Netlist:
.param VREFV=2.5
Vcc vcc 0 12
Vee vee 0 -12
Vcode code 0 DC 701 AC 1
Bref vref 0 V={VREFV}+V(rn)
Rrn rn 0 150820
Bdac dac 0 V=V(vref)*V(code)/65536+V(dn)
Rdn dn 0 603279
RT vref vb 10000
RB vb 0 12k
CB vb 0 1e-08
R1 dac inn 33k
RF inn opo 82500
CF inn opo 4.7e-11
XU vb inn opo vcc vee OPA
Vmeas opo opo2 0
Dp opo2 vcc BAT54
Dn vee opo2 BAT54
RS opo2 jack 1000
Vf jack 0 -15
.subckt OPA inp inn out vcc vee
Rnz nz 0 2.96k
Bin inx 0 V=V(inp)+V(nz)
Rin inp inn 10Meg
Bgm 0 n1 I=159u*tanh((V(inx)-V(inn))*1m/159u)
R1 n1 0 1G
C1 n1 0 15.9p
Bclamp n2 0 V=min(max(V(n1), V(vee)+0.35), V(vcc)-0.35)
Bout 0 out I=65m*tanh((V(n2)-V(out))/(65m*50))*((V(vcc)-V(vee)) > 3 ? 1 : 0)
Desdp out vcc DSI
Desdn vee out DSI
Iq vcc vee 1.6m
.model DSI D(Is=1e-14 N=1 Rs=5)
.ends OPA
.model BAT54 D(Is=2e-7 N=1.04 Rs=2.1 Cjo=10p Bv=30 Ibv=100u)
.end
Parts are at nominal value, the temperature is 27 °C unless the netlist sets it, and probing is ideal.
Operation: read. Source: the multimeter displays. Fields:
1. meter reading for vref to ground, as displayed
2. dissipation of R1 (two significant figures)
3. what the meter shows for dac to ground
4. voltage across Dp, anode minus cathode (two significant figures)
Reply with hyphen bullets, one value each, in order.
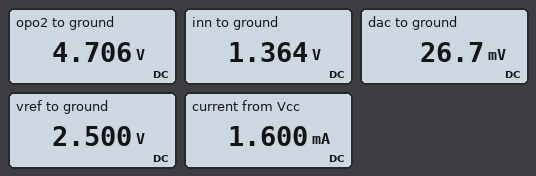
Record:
- 2.500 V
- 54 µW
- 26.7 mV
- -7.3 V
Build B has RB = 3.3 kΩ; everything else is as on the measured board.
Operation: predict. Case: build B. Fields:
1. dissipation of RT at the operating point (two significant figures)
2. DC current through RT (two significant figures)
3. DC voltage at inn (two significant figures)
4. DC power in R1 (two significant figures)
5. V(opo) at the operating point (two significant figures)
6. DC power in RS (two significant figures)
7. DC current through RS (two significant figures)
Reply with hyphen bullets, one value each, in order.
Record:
- 350 µW
- 190 µA
- 620 mV
- 11 µW
- 2.1 V
- 290 mW
- 17 mA
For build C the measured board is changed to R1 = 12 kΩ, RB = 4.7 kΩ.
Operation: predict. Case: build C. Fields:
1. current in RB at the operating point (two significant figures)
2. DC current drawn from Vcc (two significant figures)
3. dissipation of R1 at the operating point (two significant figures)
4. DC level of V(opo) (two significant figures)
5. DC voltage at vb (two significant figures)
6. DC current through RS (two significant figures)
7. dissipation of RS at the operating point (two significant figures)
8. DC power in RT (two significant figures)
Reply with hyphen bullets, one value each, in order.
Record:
- 170 µA
- 1.6 mA
- 50 µW
- 6.1 V
- 800 mV
- 21 mA
- 450 mW
- 290 µW
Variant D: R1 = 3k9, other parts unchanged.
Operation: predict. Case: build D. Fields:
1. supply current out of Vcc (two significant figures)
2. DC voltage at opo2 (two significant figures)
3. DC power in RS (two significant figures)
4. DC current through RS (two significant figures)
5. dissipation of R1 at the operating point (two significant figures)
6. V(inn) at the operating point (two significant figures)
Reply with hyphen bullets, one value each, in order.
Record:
- 1.6 mA
- 10 V
- 640 mW
- 25 mA
- 55 µW
- 490 mV
